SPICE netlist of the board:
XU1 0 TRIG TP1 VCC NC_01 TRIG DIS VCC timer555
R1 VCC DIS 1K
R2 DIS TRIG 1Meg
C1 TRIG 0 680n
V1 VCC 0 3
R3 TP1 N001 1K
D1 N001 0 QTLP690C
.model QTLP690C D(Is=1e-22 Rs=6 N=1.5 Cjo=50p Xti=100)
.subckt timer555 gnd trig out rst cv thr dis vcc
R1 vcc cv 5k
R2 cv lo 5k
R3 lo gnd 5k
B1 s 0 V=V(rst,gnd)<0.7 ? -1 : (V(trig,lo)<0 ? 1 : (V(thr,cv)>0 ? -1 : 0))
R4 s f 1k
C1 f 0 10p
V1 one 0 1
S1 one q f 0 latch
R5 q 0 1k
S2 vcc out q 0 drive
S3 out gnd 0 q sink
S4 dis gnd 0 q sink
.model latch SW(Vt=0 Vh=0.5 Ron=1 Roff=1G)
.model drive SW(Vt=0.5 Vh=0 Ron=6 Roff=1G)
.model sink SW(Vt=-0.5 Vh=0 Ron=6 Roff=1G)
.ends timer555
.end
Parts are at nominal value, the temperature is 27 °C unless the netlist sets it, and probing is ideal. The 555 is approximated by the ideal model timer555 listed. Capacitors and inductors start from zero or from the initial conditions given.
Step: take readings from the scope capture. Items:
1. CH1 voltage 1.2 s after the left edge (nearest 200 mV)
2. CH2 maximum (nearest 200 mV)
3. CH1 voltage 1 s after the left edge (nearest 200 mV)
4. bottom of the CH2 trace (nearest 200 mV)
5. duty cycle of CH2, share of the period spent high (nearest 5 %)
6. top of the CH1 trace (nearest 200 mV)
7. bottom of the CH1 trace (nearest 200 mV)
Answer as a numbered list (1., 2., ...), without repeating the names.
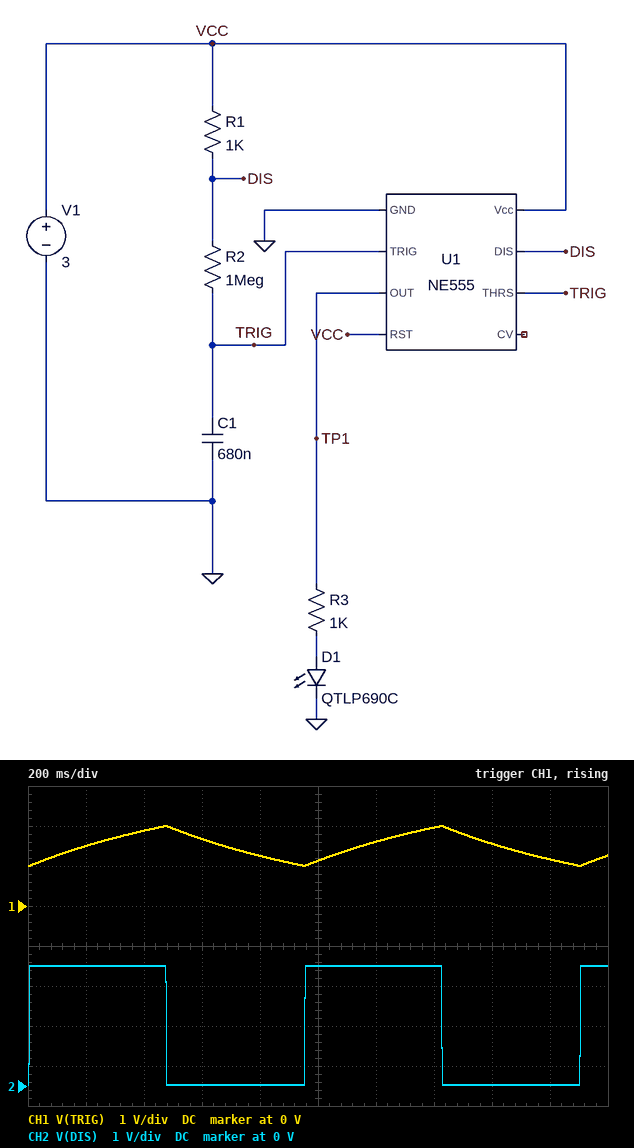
1. 1.6 V
2. 3.0 V
3. 1.2 V
4. 0 V
5. 50 %
6. 2.0 V
7. 1.0 V
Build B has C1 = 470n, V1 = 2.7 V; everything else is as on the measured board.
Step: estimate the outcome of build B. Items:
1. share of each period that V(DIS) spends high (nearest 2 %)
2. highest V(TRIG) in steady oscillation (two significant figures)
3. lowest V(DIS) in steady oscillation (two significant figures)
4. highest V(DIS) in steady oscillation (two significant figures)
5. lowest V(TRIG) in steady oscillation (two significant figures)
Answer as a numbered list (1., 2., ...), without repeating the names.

1. 50 %
2. 1.8 V
3. 16 mV
4. 2.7 V
5. 900 mV
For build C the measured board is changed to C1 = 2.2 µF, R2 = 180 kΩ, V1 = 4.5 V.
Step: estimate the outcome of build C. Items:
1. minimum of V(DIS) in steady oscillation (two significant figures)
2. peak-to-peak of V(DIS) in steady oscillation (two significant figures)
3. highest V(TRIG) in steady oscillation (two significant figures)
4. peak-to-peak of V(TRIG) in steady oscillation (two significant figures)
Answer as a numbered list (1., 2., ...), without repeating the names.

1. 27 mV
2. 4.5 V
3. 3.0 V
4. 1.5 V
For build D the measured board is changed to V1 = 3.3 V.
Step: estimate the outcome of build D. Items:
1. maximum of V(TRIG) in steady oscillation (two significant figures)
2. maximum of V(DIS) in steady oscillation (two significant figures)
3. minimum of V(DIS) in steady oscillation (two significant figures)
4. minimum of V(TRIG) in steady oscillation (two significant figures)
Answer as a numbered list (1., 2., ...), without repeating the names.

1. 2.2 V
2. 3.3 V
3. 20 mV
4. 1.1 V
